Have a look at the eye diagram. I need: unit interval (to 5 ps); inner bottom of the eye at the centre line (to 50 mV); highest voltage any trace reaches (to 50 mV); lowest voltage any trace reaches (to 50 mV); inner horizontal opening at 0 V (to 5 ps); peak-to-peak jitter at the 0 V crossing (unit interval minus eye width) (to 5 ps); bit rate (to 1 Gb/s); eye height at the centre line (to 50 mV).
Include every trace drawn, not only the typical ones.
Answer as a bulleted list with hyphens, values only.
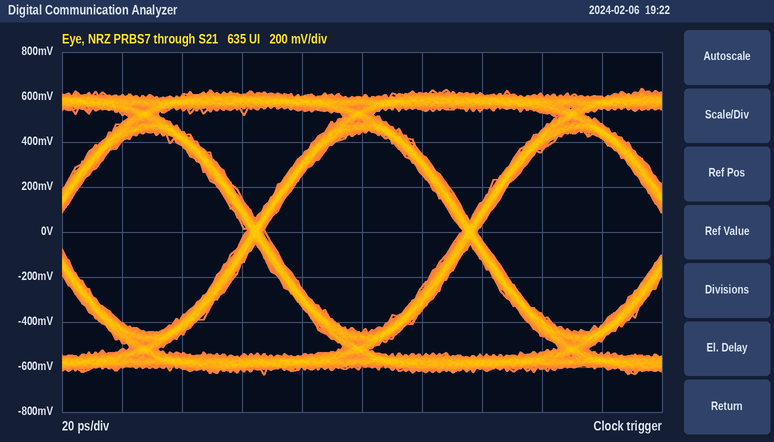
- 70 ps
- -450 mV
- 650 mV
- -650 mV
- 65 ps
- 5 ps
- 14 Gb/s
- 900 mV
